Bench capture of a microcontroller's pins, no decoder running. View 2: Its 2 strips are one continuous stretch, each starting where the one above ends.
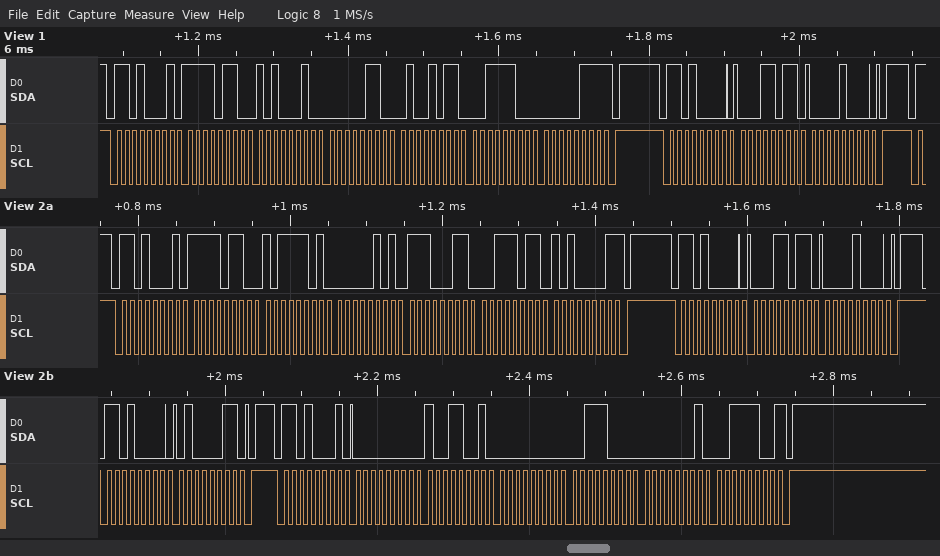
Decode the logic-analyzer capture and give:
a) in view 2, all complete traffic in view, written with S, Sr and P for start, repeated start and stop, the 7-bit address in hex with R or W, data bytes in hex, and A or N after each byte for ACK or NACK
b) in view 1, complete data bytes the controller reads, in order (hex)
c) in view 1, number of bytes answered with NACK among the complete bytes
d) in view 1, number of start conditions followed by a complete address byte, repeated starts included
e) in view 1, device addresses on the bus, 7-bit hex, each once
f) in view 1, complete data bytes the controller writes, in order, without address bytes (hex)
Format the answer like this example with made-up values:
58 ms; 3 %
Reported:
S 68R A F6 A BD A 05 A E3 A 3B A A1 N P S 68W A 1B A 08 A P S 68W A 43 A P S 68R A 00 A 99 A 00 A 38 A 01 A 3C N P; F6 A2 06 4B 3C 07; 1; 2; 0x68; 1B 08
